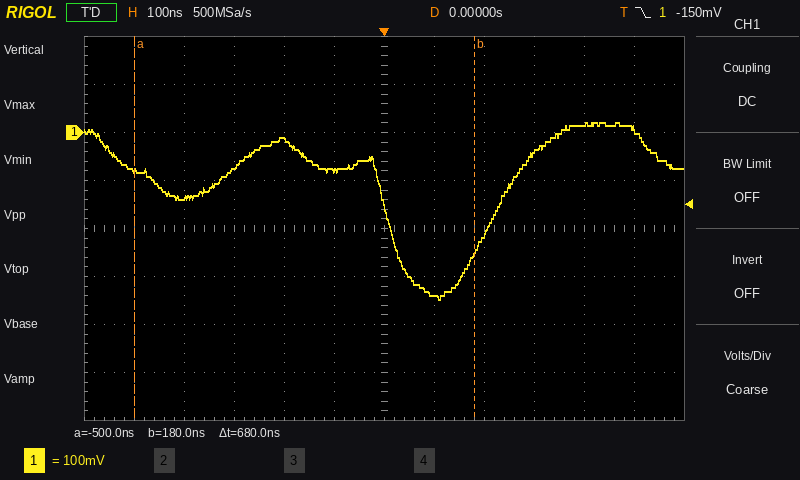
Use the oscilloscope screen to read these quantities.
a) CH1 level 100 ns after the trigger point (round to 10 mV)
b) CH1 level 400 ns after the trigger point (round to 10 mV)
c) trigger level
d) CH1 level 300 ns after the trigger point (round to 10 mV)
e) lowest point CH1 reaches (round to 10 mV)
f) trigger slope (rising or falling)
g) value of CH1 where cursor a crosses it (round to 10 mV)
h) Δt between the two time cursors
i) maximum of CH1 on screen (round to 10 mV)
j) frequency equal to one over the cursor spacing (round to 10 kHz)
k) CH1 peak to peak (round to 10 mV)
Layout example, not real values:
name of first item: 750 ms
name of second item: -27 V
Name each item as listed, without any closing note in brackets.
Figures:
CH1 level 100 ns after the trigger point: -340 mV
CH1 level 400 ns after the trigger point: 20 mV
trigger level: -150 mV
CH1 level 300 ns after the trigger point: -40 mV
lowest point CH1 reaches: -350 mV
trigger slope: falling
value of CH1 where cursor a crosses it: -80 mV
Δt between the two time cursors: 680 ns
maximum of CH1 on screen: 20 mV
frequency equal to one over the cursor spacing: 1.47 MHz
CH1 peak to peak: 370 mV
